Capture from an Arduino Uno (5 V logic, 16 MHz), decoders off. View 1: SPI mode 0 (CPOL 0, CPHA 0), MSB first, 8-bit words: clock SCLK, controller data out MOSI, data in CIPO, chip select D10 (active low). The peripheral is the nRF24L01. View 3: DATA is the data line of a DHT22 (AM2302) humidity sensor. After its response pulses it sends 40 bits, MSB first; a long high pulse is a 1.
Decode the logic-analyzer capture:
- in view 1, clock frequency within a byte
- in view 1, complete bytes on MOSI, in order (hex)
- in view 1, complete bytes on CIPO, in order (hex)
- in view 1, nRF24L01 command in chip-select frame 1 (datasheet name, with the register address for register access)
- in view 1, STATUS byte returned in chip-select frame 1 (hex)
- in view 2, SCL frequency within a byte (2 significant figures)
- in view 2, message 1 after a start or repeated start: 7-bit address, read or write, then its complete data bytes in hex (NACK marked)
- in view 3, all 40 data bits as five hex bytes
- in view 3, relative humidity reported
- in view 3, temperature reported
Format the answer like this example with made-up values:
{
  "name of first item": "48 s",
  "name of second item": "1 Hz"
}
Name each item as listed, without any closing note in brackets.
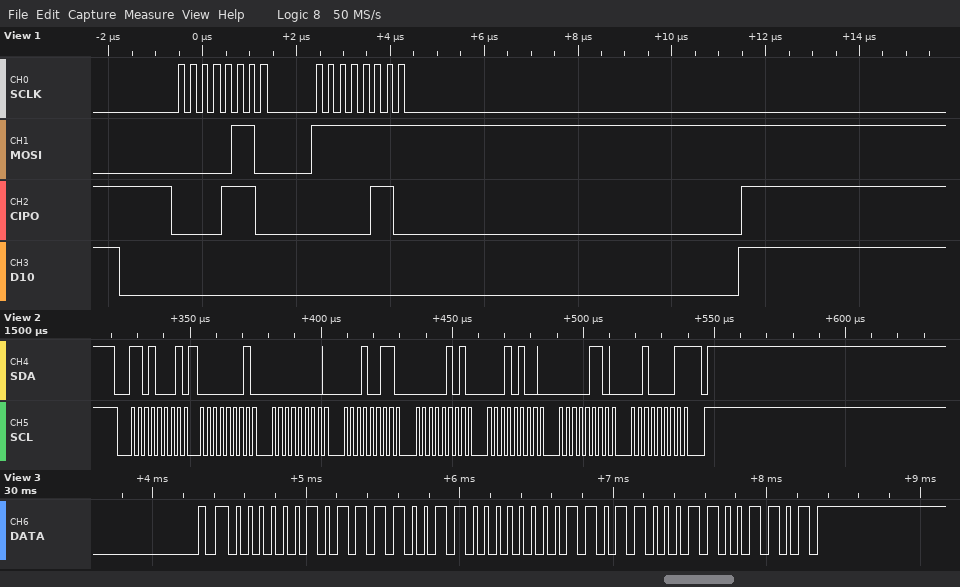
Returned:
{
  "in view 1, clock frequency within a byte": "4 MHz",
  "in view 1, complete bytes on MOSI, in order": "06 FF",
  "in view 1, complete bytes on CIPO, in order": "0E 06",
  "in view 1, nRF24L01 command in chip-select frame 1": "R_REGISTER 0x06",
  "in view 1, STATUS byte returned in chip-select frame 1": "0x0E",
  "in view 2, SCL frequency within a byte": "400 kHz",
  "in view 2, message 1 after a start or repeated start: 7-bit address, read or write, then its complete data bytes in hex": "0x68 read: 01 00 13 05 14 06 21 NACK",
  "in view 3, all 40 data bits as five hex bytes": "02 F3 00 D8 CD",
  "in view 3, relative humidity reported": "75.5 %",
  "in view 3, temperature reported": "21.6 °C"
}
